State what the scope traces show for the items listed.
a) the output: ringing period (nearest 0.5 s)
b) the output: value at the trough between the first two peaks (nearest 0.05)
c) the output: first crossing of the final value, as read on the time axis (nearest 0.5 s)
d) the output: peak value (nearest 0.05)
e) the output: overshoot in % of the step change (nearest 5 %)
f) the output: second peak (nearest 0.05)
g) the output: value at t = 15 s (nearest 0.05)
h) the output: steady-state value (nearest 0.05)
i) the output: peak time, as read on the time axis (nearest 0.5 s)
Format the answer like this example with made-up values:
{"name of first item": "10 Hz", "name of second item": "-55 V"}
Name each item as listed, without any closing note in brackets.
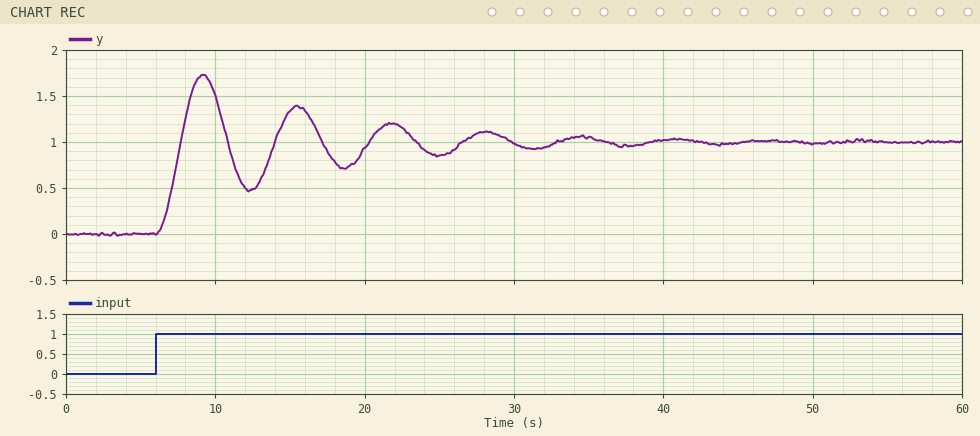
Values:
{"the output: ringing period": "6.5 s", "the output: value at the trough between the first two peaks": "0.45", "the output: first crossing of the final value, as read on the time axis": "7.5 s", "the output: peak value": "1.75", "the output: overshoot in % of the step change": "75 %", "the output: second peak": "1.40", "the output: value at t = 15 s": "1.35", "the output: steady-state value": "1.00", "the output: peak time, as read on the time axis": "9.0 s"}
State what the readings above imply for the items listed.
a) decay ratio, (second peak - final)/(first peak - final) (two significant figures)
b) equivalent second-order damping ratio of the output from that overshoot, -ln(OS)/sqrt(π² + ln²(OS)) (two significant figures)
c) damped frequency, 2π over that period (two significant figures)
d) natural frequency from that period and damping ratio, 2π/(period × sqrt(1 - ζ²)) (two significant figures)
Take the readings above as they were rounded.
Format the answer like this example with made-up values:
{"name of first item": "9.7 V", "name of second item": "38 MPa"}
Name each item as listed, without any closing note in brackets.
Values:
{"decay ratio, (second peak - final)/(first peak - final)": "0.53", "equivalent second-order damping ratio of the output from that overshoot, -ln(OS)/sqrt(π² + ln²(OS))": "0.091", "damped frequency, 2π over that period": "0.97 rad/s", "natural frequency from that period and damping ratio, 2π/(period × sqrt(1 - ζ²))": "0.97 rad/s"}
